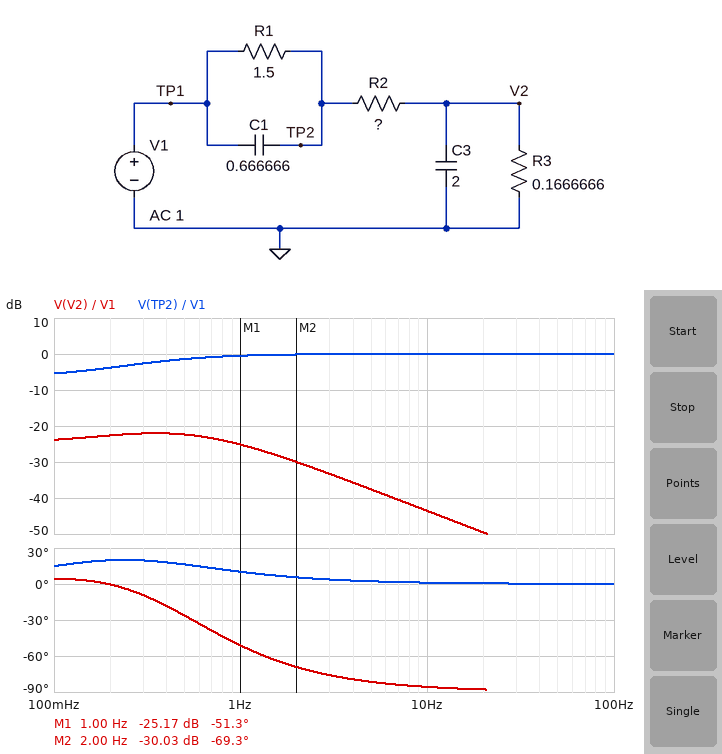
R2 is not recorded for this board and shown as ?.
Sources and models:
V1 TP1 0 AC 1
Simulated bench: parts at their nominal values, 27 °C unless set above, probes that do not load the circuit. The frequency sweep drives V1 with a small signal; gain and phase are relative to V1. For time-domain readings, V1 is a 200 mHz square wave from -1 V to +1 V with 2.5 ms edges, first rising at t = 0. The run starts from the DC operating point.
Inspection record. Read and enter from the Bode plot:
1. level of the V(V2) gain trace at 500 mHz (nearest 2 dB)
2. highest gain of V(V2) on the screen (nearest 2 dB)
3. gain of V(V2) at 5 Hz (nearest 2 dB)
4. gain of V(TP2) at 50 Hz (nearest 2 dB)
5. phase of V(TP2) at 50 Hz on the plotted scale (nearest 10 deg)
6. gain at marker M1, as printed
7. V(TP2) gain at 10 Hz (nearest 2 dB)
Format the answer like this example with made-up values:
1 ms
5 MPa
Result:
-22 dB
-22 dB
-38 dB
0 dB
0 deg
-25.17 dB
0 dB
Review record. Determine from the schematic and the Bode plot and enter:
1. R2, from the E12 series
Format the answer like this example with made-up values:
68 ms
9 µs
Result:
1.2 Ω
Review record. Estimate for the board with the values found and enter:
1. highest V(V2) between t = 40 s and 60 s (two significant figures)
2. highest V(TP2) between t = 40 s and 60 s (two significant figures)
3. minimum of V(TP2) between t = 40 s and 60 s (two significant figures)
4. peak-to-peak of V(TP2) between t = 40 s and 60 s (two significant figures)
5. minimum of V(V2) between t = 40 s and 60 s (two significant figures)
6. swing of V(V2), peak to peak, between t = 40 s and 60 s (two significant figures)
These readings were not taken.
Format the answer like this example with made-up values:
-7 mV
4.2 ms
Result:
91 mV
1.5 V
-1.5 V
3.0 V
-91 mV
180 mV
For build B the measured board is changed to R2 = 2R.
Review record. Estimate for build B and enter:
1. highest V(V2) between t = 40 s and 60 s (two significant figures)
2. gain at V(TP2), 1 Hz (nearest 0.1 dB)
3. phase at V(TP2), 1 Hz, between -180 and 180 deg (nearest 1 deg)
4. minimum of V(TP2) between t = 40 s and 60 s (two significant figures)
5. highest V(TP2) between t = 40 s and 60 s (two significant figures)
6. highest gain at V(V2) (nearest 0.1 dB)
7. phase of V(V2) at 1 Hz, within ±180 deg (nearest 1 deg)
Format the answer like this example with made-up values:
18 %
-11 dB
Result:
62 mV
-0.2 dB
6 deg
-1.4 V
1.4 V
-25.1 dB
-56 deg
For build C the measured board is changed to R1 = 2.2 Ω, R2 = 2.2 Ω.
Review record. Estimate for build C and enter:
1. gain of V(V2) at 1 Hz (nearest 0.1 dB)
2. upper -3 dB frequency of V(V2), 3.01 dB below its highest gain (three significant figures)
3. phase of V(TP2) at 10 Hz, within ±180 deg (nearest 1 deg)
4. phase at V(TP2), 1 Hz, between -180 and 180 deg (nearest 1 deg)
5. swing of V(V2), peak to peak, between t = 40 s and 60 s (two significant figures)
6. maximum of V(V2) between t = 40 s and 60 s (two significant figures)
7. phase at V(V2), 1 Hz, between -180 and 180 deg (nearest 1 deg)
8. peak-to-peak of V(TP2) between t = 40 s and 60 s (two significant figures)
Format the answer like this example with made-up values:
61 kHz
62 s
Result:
-30.0 dB
792 mHz
1 deg
6 deg
120 mV
60 mV
-57 deg
2.9 V
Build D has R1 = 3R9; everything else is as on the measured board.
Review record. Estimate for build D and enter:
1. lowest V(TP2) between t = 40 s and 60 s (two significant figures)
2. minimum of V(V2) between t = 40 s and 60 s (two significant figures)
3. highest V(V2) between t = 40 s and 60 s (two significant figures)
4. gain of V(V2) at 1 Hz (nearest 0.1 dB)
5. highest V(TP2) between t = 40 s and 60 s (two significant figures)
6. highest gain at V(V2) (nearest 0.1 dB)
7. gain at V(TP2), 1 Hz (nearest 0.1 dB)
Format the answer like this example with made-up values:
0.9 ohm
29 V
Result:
-1.7 V
-110 mV
110 mV
-25.0 dB
1.7 V
-21.5 dB
-0.3 dB
